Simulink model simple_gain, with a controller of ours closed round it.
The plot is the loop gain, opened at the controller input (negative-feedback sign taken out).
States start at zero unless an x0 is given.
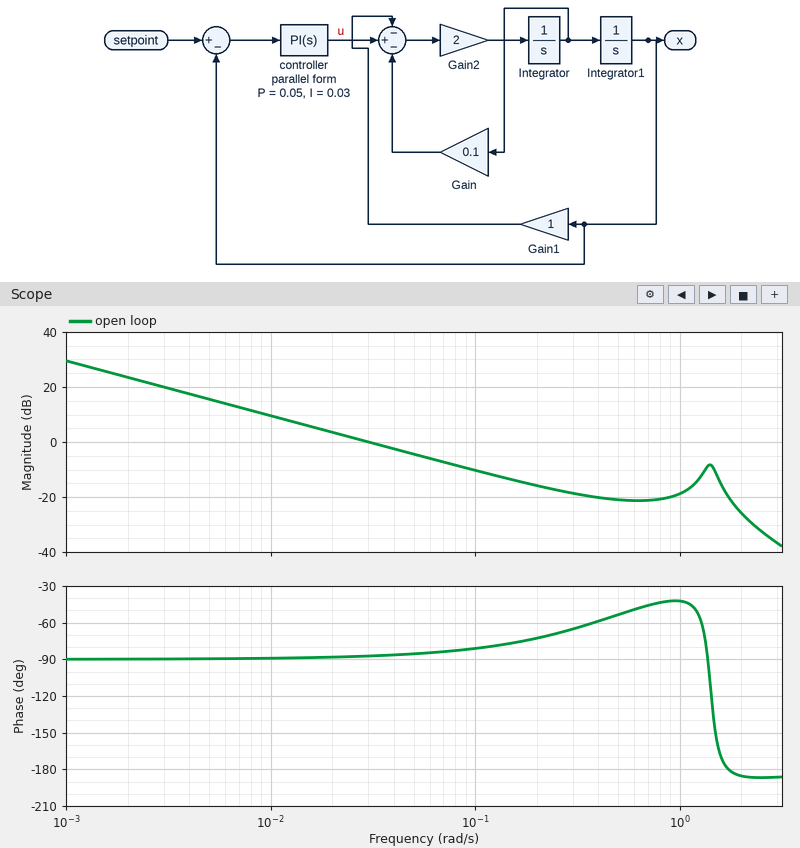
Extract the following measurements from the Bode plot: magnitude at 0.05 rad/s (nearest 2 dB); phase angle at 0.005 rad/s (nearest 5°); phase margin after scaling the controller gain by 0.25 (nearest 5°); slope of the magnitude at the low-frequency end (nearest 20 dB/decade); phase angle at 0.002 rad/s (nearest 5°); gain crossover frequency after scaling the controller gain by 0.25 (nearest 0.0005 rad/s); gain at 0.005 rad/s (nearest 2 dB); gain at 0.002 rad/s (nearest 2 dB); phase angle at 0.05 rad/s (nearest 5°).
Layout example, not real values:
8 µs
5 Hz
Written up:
-4 dB
-90°
90°
-20 dB/decade
-90°
0.0075 rad/s
16 dB
24 dB
-85°
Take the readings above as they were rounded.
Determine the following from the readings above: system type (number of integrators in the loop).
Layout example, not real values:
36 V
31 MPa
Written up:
1
